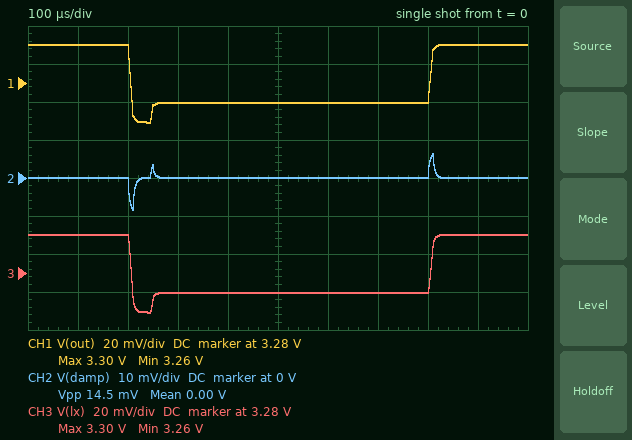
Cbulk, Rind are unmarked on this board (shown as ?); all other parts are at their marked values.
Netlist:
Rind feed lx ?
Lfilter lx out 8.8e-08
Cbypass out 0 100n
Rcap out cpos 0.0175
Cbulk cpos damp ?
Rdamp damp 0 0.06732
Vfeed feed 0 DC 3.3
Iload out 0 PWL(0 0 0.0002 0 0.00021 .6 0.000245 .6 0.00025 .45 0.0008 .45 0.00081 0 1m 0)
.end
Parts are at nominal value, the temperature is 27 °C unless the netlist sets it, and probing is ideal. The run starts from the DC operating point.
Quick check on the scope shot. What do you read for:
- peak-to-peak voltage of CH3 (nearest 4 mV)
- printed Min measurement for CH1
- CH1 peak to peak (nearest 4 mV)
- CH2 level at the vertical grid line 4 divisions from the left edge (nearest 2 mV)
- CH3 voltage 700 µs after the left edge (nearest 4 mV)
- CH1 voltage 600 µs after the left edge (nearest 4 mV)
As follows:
40 mV
3.26 V
40 mV
0 V
3.268 V
3.268 V
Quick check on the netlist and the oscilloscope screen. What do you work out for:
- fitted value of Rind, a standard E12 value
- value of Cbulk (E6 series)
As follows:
0.068 Ω
33 µF
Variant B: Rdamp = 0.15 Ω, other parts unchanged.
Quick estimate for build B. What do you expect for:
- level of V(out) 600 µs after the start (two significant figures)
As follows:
3.3 V
